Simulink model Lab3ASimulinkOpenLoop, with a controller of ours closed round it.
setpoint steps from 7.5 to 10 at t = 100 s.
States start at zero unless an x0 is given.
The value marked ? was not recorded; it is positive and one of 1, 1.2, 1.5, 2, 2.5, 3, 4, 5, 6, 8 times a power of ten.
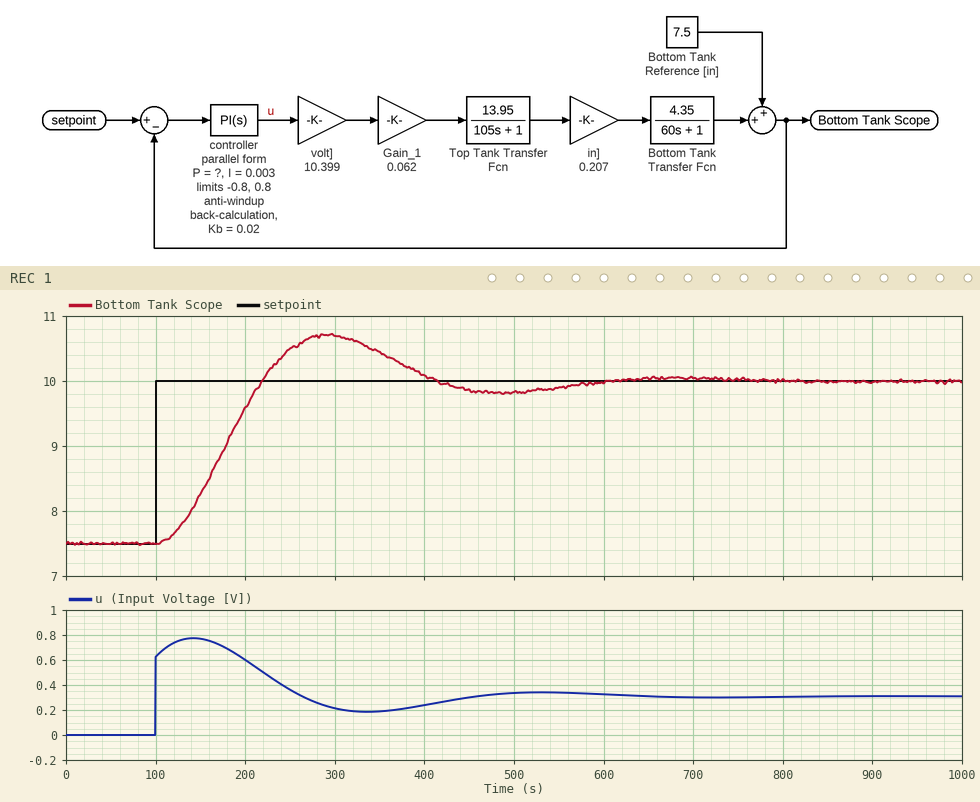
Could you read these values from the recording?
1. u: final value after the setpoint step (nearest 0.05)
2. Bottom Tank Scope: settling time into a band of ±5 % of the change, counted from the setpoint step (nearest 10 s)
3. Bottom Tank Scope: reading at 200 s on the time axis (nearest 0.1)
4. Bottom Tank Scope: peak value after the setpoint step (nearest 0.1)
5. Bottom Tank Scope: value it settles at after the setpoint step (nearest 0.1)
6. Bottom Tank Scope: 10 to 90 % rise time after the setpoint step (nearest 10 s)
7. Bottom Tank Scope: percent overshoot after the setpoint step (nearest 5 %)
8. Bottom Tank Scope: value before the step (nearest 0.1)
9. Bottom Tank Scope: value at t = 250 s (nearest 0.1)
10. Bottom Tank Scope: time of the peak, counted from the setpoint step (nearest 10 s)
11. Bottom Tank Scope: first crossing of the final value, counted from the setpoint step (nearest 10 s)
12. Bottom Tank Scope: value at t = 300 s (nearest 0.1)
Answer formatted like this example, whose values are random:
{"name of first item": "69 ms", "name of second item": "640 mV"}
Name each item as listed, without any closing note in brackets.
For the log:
{"u: final value after the setpoint step": "0.30", "Bottom Tank Scope: settling time into a band of ±5 % of the change, counted from the setpoint step": "440 s", "Bottom Tank Scope: reading at 200 s on the time axis": "9.6", "Bottom Tank Scope: peak value after the setpoint step": "10.7", "Bottom Tank Scope: value it settles at after the setpoint step": "10.0", "Bottom Tank Scope: 10 to 90 % rise time after the setpoint step": "80 s", "Bottom Tank Scope: percent overshoot after the setpoint step": "30 %", "Bottom Tank Scope: value before the step": "7.5", "Bottom Tank Scope: value at t = 250 s": "10.5", "Bottom Tank Scope: time of the peak, counted from the setpoint step": "190 s", "Bottom Tank Scope: first crossing of the final value, counted from the setpoint step": "120 s", "Bottom Tank Scope: value at t = 300 s": "10.7"}
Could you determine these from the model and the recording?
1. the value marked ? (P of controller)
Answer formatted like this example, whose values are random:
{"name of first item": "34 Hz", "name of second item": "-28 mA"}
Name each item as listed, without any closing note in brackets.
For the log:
{"the value marked ?": "0.25"}
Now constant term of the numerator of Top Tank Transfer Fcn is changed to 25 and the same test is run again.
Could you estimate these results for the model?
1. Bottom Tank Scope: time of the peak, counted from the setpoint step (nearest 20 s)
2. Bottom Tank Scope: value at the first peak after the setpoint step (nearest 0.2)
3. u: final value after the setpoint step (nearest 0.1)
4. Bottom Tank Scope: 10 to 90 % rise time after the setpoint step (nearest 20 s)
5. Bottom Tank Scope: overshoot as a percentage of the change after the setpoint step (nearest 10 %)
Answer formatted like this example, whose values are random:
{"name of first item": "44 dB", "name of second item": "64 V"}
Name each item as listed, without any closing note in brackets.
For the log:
{"Bottom Tank Scope: time of the peak, counted from the setpoint step": "140 s", "Bottom Tank Scope: value at the first peak after the setpoint step": "11.0", "u: final value after the setpoint step": "0.2", "Bottom Tank Scope: 10 to 90 % rise time after the setpoint step": "60 s", "Bottom Tank Scope: overshoot as a percentage of the change after the setpoint step": "40 %"}
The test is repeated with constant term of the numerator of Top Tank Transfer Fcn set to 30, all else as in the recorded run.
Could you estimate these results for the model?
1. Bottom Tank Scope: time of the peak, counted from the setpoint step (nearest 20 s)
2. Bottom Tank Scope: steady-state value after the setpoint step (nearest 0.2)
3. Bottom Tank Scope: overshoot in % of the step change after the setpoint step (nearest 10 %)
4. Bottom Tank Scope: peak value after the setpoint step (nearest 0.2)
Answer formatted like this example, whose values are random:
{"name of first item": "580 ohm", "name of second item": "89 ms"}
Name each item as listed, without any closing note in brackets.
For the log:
{"Bottom Tank Scope: time of the peak, counted from the setpoint step": "120 s", "Bottom Tank Scope: steady-state value after the setpoint step": "10.0", "Bottom Tank Scope: overshoot in % of the step change after the setpoint step": "40 %", "Bottom Tank Scope: peak value after the setpoint step": "11.0"}
